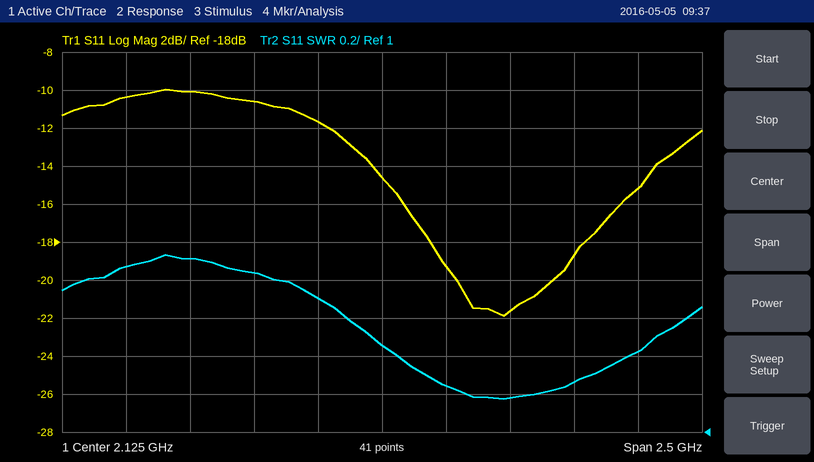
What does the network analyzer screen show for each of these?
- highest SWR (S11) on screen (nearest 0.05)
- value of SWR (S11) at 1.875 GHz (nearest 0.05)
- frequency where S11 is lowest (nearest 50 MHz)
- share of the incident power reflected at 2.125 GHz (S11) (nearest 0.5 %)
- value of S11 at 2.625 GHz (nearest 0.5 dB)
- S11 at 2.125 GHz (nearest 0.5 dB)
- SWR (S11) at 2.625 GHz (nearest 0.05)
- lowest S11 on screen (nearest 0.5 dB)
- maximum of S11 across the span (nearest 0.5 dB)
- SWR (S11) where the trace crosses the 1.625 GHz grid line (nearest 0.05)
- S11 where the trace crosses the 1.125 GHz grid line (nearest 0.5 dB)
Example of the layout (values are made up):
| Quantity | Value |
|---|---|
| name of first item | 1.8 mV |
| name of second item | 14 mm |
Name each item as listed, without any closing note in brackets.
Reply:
| Quantity | Value |
|---|---|
| highest SWR (S11) on screen | 1.95 |
| value of SWR (S11) at 1.875 GHz | 1.70 |
| frequency where S11 is lowest | 2.60 GHz |
| share of the incident power reflected at 2.125 GHz (S11) | 3.5 % |
| value of S11 at 2.625 GHz | -21.5 dB |
| S11 at 2.125 GHz | -14.5 dB |
| SWR (S11) at 2.625 GHz | 1.20 |
| lowest S11 on screen | -22.0 dB |
| maximum of S11 across the span | -10.0 dB |
| SWR (S11) where the trace crosses the 1.625 GHz grid line | 1.85 |
| S11 where the trace crosses the 1.125 GHz grid line | -10.5 dB |
